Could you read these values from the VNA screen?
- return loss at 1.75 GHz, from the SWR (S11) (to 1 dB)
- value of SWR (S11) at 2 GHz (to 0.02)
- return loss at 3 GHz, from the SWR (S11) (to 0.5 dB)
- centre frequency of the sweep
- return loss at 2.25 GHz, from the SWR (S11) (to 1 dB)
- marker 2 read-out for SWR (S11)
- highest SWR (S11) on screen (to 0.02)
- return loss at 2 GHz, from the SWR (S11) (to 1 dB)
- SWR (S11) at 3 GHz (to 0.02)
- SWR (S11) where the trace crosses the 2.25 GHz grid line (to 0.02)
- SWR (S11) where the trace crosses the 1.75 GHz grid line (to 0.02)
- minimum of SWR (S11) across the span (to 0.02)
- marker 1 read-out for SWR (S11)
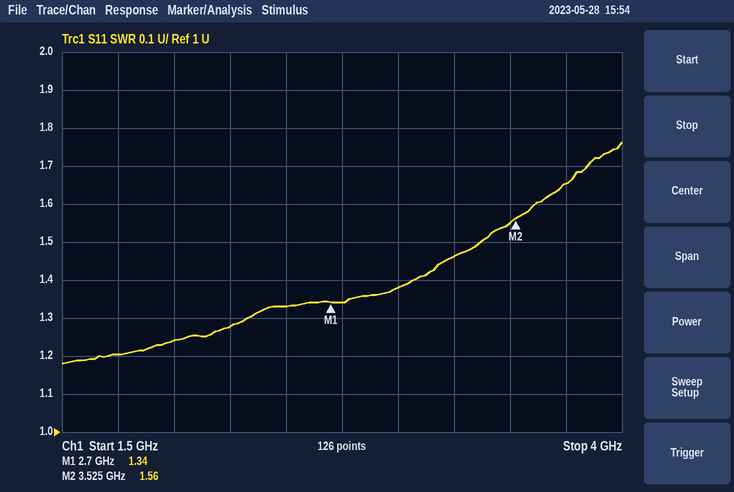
21 dB
1.24
16.0 dB
2.75 GHz
18 dB
1.56
1.76
19 dB
1.38
1.28
1.20
1.18
1.34
